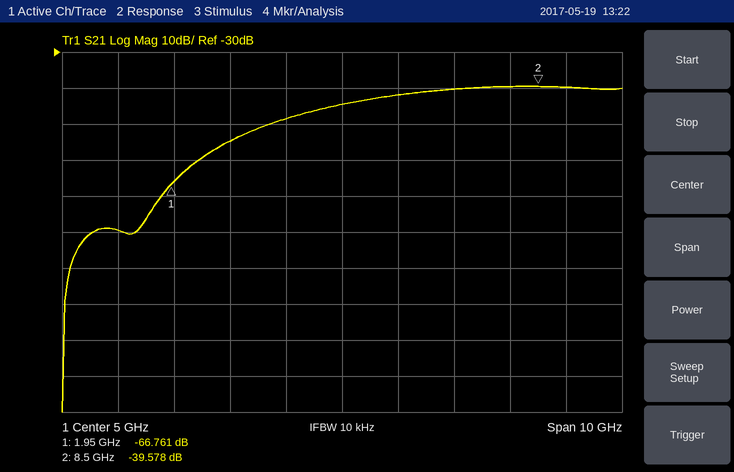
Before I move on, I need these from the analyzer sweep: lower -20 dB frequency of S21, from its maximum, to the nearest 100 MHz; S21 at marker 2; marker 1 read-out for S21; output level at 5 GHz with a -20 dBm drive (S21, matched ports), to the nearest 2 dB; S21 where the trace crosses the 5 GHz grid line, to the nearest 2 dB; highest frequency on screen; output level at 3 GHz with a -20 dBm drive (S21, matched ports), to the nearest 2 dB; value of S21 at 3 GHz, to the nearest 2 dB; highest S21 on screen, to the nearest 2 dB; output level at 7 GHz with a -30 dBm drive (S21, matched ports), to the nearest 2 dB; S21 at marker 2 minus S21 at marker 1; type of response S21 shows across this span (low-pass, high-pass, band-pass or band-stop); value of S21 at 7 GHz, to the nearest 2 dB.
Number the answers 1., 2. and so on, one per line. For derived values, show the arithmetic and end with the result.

1. 2.5 GHz
2. -39.578 dB
3. -66.761 dB
4. -20 dBm + (-44 dB) = -64 dBm
5. -44 dB
6. 10 GHz
7. -20 dBm + (-54 dB) = -74 dBm
8. -54 dB
9. -40 dB
10. -30 dBm + (-40 dB) = -70 dBm
11. -39.578 − (-66.761) = 27.183 dB
12. high-pass
13. -40 dB
